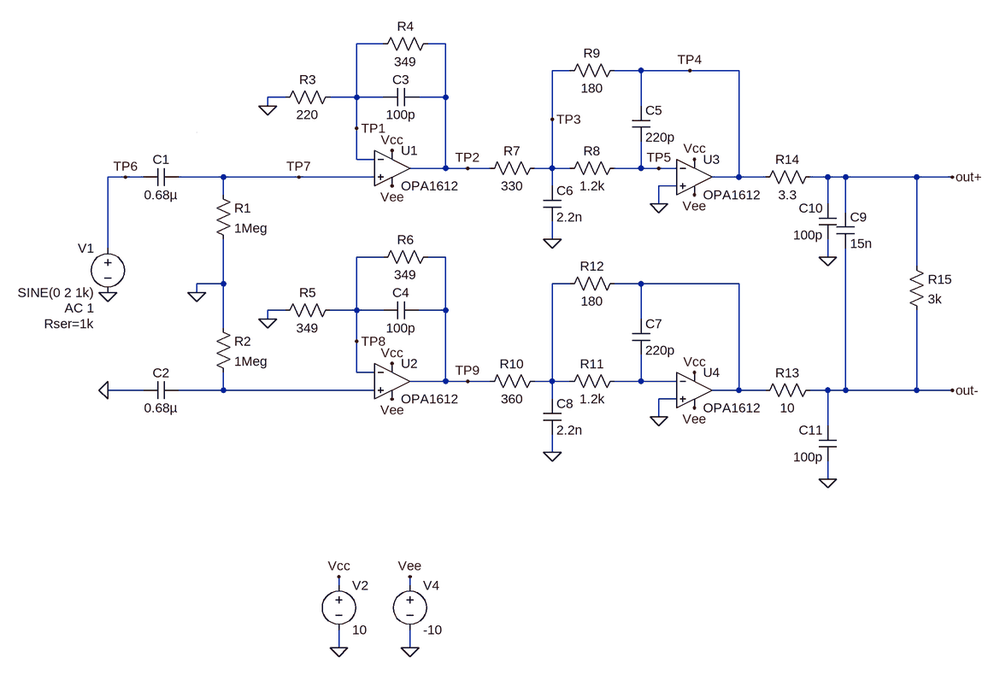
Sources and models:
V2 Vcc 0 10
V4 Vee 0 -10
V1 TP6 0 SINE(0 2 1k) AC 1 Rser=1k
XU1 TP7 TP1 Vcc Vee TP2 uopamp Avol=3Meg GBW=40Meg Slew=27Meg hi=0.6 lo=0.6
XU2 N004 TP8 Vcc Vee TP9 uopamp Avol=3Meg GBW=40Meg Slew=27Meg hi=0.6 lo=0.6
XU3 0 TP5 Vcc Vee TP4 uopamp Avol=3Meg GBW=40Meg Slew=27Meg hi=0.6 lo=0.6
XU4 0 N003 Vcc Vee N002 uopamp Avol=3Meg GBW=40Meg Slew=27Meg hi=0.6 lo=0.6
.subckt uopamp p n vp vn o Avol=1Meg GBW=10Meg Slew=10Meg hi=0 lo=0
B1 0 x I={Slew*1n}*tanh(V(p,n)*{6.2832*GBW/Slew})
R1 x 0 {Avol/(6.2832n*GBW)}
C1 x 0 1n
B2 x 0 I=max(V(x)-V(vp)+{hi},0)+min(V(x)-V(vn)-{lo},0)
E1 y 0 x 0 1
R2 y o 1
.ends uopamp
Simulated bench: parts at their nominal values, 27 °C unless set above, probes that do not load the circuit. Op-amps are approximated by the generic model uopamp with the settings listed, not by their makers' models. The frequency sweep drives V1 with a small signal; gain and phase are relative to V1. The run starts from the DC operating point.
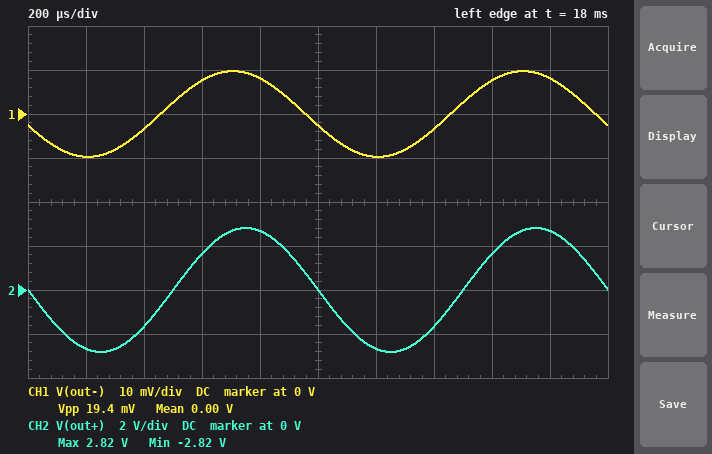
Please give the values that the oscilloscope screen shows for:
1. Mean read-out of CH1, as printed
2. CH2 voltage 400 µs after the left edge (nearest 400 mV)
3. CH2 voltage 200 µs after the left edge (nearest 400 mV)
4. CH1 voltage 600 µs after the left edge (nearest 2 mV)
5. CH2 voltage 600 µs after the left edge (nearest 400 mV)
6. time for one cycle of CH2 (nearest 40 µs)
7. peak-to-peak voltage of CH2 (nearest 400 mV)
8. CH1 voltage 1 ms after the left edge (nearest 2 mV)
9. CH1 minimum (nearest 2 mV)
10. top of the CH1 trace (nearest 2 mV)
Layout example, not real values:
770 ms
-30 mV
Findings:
0.00 V
-1.6 V
-2.8 V
8 mV
1.6 V
1.00 ms
5.6 V
-2 mV
-10 mV
10 mV
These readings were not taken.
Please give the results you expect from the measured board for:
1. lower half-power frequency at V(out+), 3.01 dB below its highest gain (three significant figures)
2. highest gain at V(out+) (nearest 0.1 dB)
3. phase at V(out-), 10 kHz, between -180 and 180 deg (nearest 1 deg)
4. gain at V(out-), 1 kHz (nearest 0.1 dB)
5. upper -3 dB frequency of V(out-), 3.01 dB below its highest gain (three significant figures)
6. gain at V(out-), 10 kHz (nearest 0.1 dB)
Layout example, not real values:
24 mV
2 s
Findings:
234 mHz
3.0 dB
-112 deg
-46.3 dB
745 kHz
-37.1 dB
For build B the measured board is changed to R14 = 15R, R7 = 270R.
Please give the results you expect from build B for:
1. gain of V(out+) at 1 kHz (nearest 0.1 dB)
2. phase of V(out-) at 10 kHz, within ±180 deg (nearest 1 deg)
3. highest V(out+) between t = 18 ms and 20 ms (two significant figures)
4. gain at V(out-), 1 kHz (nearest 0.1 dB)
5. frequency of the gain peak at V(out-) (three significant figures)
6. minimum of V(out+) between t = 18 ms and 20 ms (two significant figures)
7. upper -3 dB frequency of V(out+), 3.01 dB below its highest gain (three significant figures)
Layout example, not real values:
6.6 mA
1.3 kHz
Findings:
4.7 dB
-113 deg
3.4 V
-44.6 dB
376 kHz
-3.4 V
342 kHz
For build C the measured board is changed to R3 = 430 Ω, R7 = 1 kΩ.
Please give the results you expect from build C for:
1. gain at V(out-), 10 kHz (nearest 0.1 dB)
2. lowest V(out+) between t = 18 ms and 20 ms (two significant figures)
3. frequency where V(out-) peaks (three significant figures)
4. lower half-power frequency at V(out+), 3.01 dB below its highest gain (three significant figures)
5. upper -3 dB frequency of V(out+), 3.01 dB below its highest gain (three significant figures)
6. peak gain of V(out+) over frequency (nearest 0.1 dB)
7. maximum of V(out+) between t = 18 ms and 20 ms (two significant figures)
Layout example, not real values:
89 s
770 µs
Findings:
-49.8 dB
-650 mV
454 kHz
269 mHz
543 kHz
-9.2 dB
650 mV
